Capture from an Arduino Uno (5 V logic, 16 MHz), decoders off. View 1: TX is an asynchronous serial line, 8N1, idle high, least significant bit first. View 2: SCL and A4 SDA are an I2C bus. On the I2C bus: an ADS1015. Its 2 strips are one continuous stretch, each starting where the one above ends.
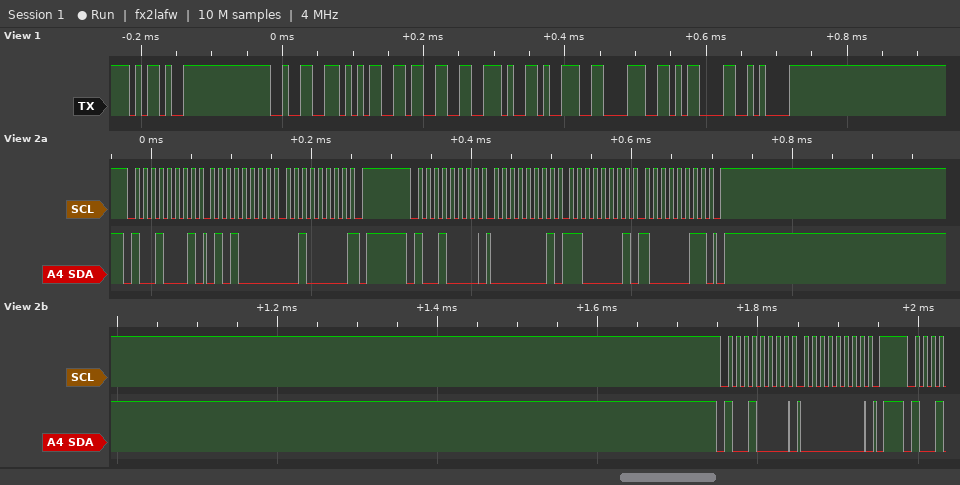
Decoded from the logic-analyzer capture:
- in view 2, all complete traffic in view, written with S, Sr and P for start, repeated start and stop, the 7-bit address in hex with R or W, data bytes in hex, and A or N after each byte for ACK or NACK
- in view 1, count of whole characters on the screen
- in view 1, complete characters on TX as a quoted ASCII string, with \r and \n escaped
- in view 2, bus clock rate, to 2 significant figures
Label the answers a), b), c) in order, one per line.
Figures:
a) S 48R A 50 A 20 N P S 48W A 01 A C1 A 83 A P S 48W A 00 A P
b) 9
c) "-253.98\r\n"
d) 100 kHz
